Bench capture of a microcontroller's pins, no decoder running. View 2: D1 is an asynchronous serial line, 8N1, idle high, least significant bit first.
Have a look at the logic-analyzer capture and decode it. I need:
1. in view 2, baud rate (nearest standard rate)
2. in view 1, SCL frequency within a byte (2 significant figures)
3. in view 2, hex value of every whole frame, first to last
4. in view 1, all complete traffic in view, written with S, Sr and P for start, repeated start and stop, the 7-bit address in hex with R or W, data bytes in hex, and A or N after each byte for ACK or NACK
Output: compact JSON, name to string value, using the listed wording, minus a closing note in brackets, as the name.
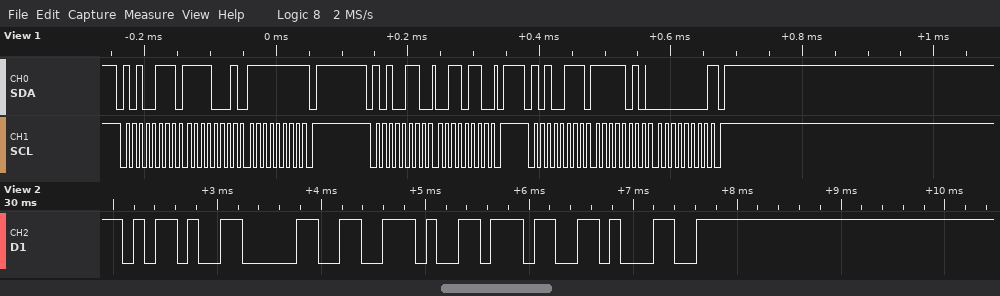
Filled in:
{"in view 2, baud rate": "9600 baud", "in view 1, SCL frequency within a byte": "100 kHz", "in view 2, hex value of every whole frame, first to last": "2D 30 2E 37 31", "in view 1, all complete traffic in view, written with S, Sr and P for start, repeated start and stop, the 7-bit address in hex with R or W, data bytes in hex, and A or N after each byte for ACK or NACK": "S 53R A F1 A FF N P S 53W A 36 A P S 53R A FA A 00 N P"}
